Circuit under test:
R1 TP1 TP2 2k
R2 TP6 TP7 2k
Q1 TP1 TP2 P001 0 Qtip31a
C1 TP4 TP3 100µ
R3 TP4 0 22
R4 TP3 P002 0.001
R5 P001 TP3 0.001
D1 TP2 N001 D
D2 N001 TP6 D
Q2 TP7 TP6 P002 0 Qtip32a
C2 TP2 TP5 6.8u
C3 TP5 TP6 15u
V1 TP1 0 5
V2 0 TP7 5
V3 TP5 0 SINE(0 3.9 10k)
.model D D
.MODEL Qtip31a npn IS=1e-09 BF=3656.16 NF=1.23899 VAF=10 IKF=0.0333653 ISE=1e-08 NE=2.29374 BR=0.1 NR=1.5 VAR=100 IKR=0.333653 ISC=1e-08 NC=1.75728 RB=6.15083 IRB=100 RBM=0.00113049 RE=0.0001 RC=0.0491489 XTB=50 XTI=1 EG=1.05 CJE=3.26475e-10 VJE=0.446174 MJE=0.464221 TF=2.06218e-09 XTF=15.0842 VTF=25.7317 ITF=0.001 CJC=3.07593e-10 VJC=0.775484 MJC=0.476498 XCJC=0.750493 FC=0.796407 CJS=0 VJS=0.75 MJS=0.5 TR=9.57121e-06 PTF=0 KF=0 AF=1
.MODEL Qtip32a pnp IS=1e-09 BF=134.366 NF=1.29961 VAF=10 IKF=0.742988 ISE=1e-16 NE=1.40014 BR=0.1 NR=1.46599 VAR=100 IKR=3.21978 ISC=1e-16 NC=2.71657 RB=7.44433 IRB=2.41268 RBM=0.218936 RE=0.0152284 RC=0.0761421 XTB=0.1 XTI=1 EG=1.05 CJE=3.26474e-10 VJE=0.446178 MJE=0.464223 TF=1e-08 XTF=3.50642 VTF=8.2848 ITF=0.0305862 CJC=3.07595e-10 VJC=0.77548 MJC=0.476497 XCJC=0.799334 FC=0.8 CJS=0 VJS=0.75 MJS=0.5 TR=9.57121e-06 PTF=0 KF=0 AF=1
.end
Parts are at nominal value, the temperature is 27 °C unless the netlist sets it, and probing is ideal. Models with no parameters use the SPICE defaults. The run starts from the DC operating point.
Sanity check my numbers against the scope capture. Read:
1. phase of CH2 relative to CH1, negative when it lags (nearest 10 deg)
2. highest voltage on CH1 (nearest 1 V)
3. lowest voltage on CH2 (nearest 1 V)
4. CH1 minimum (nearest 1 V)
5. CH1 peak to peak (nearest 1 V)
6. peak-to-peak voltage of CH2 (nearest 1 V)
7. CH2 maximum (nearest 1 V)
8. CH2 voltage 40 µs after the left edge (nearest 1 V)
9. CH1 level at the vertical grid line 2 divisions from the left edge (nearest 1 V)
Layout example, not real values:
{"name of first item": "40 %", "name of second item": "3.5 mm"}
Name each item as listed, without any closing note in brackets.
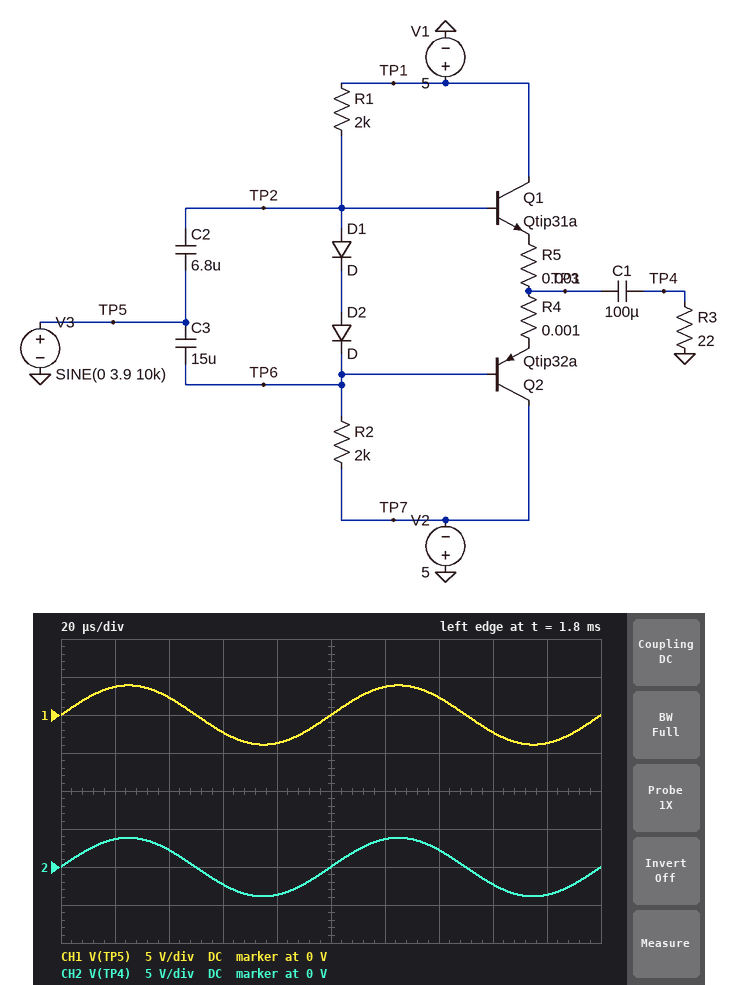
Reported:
{"phase of CH2 relative to CH1, negative when it lags": "0 deg", "highest voltage on CH1": "4 V", "lowest voltage on CH2": "-4 V", "CH1 minimum": "-4 V", "CH1 peak to peak": "8 V", "peak-to-peak voltage of CH2": "8 V", "CH2 maximum": "4 V", "CH2 voltage 40 µs after the left edge": "2 V", "CH1 level at the vertical grid line 2 divisions from the left edge": "2 V"}
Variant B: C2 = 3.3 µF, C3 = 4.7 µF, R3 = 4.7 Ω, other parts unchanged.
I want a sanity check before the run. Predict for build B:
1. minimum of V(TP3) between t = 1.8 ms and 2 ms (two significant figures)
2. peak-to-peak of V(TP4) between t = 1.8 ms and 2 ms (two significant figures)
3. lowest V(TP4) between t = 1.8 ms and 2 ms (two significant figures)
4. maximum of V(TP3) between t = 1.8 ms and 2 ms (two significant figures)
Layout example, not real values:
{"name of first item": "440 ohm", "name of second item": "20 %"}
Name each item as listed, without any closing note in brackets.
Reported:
{"minimum of V(TP3) between t = 1.8 ms and 2 ms": "-3.2 V", "peak-to-peak of V(TP4) between t = 1.8 ms and 2 ms": "7.2 V", "lowest V(TP4) between t = 1.8 ms and 2 ms": "-3.6 V", "maximum of V(TP3) between t = 1.8 ms and 2 ms": "4.0 V"}
